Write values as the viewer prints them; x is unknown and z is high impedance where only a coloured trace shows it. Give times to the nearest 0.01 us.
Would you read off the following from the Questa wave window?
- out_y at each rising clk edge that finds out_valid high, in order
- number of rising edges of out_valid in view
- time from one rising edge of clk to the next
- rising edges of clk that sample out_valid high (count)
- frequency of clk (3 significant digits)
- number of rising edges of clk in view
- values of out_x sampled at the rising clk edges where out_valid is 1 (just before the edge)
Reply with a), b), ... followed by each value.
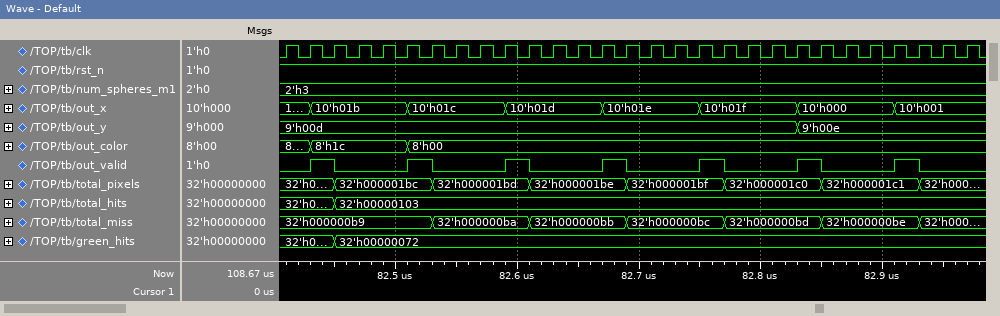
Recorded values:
a) 9'h00d, 9'h00d, 9'h00d, 9'h00d, 9'h00d, 9'h00e, 9'h00e
b) 7
c) 0.02 us
d) 7
e) 50.0 MHz
f) 29
g) 10'h01b, 10'h01c, 10'h01d, 10'h01e, 10'h01f, 10'h000, 10'h001
